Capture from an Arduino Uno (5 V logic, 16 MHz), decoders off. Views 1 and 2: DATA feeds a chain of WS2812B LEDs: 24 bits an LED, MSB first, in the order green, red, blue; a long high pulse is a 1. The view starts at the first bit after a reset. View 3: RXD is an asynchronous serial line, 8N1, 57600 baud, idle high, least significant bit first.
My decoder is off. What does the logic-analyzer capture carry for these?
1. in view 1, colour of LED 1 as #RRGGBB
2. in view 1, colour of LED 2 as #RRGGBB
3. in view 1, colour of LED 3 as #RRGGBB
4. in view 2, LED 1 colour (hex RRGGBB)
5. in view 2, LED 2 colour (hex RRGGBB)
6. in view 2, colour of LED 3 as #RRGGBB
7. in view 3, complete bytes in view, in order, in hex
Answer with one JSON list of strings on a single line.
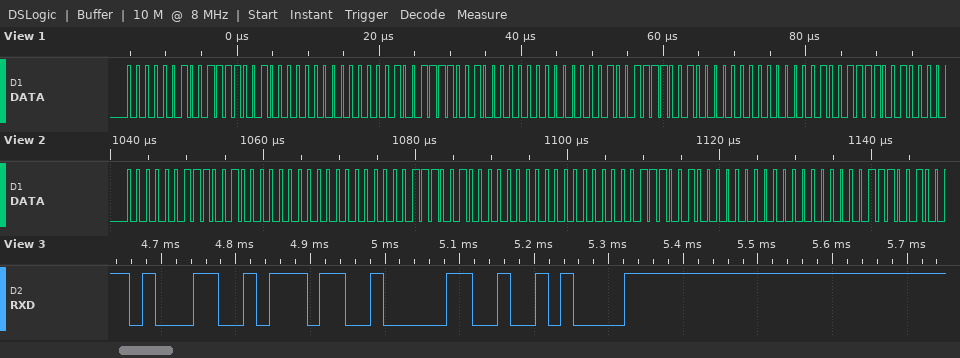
["#790200", "#790200", "#790200", "#900300", "#900300", "#900300", "31 37 30 0A"]
